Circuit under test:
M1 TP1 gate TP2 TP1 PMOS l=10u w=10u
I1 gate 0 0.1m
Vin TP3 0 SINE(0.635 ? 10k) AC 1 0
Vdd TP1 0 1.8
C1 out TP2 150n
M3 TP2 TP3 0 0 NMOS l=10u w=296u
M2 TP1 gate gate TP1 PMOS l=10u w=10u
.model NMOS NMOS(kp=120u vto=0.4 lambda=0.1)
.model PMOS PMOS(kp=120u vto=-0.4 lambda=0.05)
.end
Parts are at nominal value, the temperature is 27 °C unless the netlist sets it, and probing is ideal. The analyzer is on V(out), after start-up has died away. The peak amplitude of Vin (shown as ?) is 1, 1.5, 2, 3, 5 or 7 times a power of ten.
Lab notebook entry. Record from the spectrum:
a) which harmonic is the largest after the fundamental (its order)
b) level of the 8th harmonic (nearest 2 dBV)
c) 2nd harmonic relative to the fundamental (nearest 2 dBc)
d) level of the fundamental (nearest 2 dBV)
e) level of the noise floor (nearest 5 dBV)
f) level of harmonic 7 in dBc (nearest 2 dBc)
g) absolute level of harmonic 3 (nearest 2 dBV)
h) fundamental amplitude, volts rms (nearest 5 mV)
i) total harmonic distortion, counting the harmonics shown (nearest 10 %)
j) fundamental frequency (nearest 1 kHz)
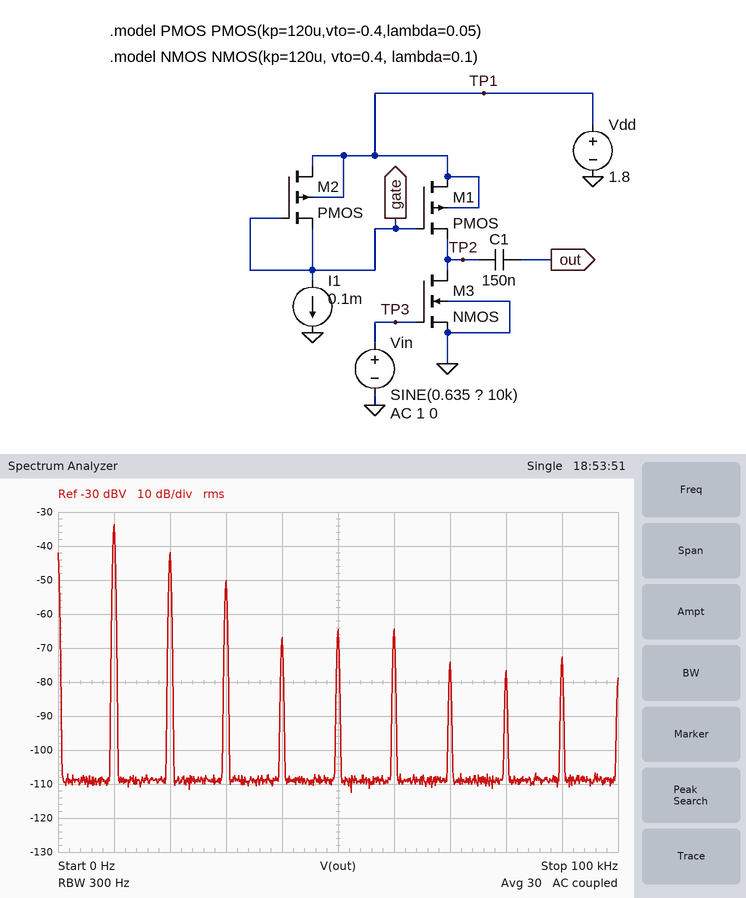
2
-76 dBV
-8 dBc
-34 dBV
-110 dBV
-40 dBc
-50 dBV
20 mV
40 %
10 kHz
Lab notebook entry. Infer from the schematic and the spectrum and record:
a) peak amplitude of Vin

1.5 mV
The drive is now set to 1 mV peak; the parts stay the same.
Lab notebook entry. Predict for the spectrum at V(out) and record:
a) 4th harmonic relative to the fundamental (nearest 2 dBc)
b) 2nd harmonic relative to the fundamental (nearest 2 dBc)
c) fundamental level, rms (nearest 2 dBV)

-24 dBc
-12 dBc
-40 dBV
